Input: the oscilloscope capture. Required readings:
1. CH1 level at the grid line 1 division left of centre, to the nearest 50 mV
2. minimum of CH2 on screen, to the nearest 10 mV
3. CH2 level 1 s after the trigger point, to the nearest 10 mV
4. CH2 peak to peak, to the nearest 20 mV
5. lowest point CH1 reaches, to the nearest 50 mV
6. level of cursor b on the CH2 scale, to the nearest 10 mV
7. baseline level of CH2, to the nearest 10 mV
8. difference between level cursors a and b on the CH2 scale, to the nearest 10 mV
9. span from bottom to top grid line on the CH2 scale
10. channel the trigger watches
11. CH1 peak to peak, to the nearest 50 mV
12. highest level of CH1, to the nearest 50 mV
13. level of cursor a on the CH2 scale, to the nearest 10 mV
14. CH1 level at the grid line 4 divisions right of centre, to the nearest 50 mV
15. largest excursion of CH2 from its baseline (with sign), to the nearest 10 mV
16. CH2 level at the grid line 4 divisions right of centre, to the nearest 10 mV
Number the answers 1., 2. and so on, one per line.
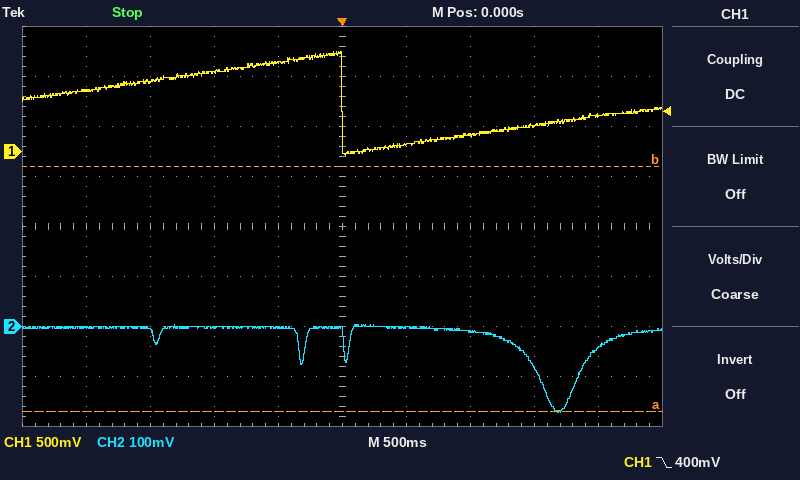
1. 900 mV
2. -170 mV
3. -10 mV
4. 180 mV
5. -50 mV
6. 320 mV
7. 0 mV
8. 490 mV
9. 800 mV
10. CH1
11. 1.05 V
12. 1.00 V
13. -170 mV
14. 350 mV
15. -170 mV
16. -40 mV
